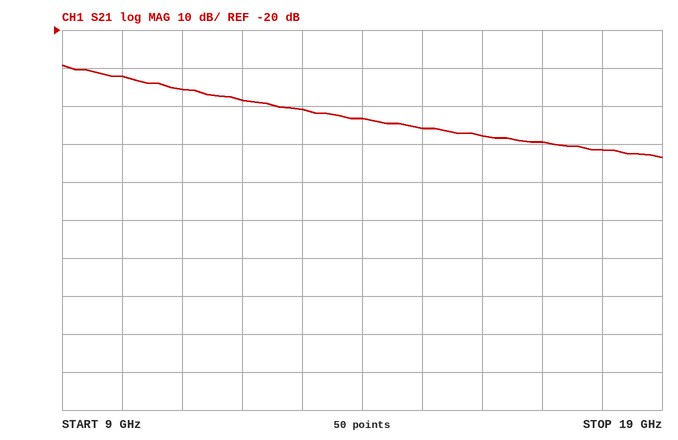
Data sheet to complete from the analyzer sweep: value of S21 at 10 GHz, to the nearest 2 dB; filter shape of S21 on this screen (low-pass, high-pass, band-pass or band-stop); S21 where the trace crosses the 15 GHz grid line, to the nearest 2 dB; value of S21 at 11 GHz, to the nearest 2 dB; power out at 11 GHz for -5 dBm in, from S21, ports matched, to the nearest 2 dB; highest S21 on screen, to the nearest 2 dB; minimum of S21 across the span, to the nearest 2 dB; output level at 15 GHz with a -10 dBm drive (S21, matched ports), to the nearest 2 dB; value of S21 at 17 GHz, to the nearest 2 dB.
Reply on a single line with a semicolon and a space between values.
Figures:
-32 dB; low-pass; -46 dB; -36 dB; -40 dBm; -30 dB; -54 dB; -56 dBm; -50 dB
